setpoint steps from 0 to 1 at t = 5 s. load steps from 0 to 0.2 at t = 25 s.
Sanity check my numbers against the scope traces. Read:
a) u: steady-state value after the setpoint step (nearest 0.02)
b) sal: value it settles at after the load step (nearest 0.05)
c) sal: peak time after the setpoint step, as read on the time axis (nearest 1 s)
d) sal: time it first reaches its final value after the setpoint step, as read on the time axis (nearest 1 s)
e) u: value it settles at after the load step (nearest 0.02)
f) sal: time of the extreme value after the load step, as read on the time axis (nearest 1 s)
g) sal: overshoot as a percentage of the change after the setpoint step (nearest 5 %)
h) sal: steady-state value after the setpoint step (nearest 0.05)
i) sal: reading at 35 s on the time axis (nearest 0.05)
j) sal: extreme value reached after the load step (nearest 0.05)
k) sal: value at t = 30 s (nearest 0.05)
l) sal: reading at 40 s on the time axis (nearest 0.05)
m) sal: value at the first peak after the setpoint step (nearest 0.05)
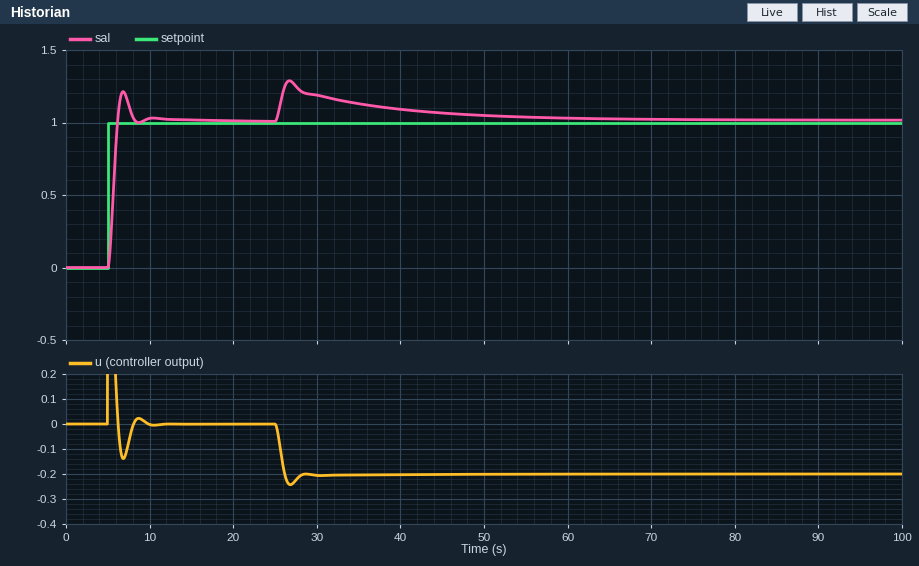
0.00
1.00
7 s
6 s
-0.20
27 s
20 %
1.00
1.15
1.30
1.20
1.10
1.20
